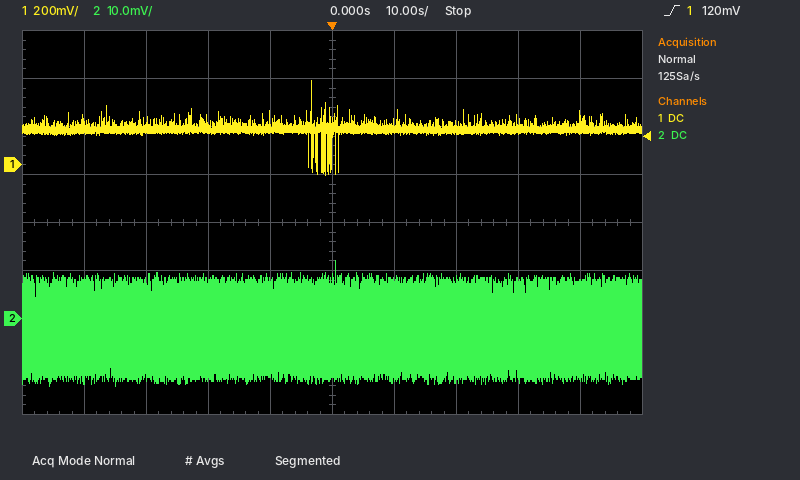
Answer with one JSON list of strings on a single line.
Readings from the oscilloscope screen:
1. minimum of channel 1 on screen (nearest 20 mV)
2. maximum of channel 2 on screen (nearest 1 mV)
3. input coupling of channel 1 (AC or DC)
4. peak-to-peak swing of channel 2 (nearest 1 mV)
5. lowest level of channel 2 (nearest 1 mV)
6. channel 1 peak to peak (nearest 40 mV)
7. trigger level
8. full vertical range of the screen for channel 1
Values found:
["-40 mV", "12 mV", "DC", "26 mV", "-14 mV", "400 mV", "120 mV", "1.6 V"]
